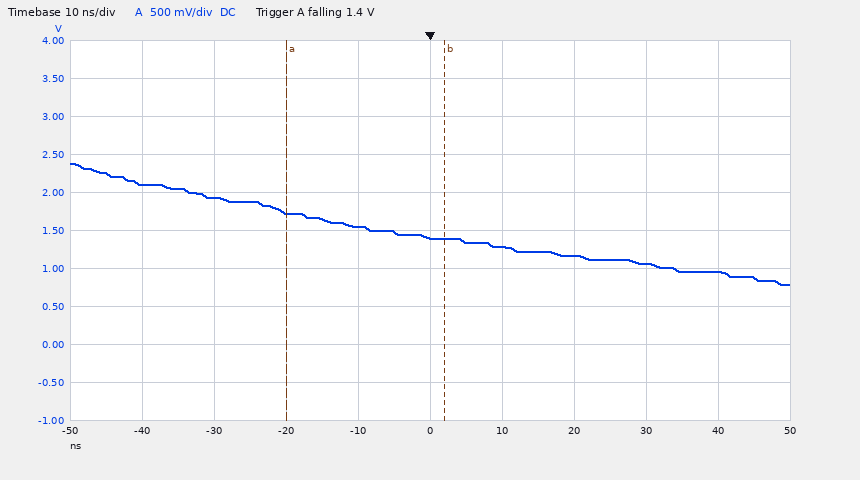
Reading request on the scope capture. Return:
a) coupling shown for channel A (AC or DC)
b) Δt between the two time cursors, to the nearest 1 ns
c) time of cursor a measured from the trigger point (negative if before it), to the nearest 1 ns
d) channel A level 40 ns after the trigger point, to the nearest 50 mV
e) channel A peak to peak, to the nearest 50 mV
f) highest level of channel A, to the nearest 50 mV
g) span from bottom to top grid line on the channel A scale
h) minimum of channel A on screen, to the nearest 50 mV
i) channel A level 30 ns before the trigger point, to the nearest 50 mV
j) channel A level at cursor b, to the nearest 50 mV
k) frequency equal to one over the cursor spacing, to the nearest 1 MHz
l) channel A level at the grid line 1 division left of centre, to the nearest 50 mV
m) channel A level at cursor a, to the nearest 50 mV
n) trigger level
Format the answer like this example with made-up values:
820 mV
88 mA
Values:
DC
22 ns
-20 ns
950 mV
1.60 V
2.40 V
5 V
800 mV
1.95 V
1.40 V
45 MHz
1.55 V
1.75 V
1.4 V
